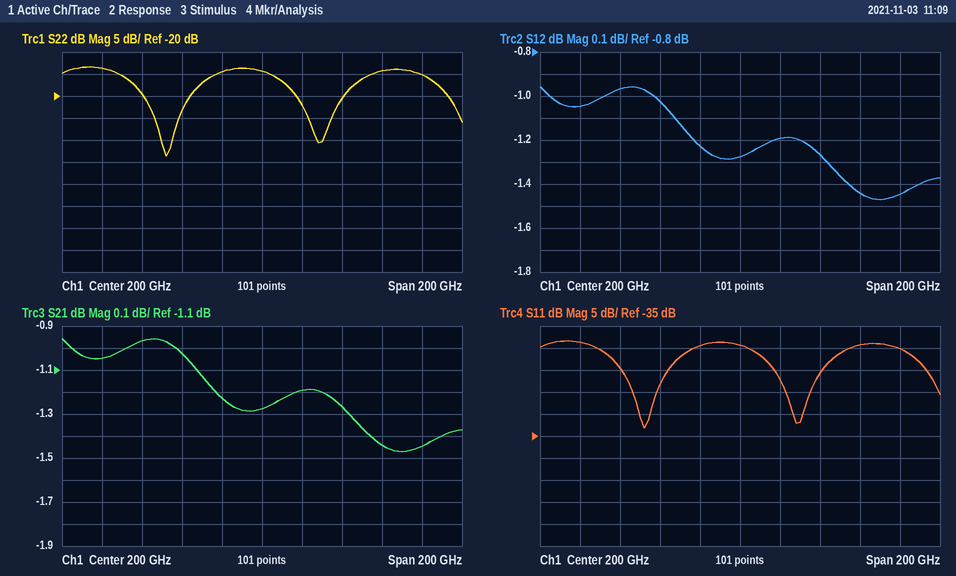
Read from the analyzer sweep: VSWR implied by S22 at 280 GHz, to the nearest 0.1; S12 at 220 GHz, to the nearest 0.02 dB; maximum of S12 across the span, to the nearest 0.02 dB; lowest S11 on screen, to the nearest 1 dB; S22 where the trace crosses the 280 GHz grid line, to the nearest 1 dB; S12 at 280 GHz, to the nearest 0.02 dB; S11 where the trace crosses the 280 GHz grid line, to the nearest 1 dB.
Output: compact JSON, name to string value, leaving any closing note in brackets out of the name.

{"VSWR implied by S22 at 280 GHz, to the nearest 0.1": "1.4", "S12 at 220 GHz, to the nearest 0.02 dB": "-1.20 dB", "maximum of S12 across the span, to the nearest 0.02 dB": "-0.96 dB", "lowest S11 on screen, to the nearest 1 dB": "-33 dB", "S22 where the trace crosses the 280 GHz grid line, to the nearest 1 dB": "-15 dB", "S12 at 280 GHz, to the nearest 0.02 dB": "-1.44 dB", "S11 where the trace crosses the 280 GHz grid line, to the nearest 1 dB": "-15 dB"}
